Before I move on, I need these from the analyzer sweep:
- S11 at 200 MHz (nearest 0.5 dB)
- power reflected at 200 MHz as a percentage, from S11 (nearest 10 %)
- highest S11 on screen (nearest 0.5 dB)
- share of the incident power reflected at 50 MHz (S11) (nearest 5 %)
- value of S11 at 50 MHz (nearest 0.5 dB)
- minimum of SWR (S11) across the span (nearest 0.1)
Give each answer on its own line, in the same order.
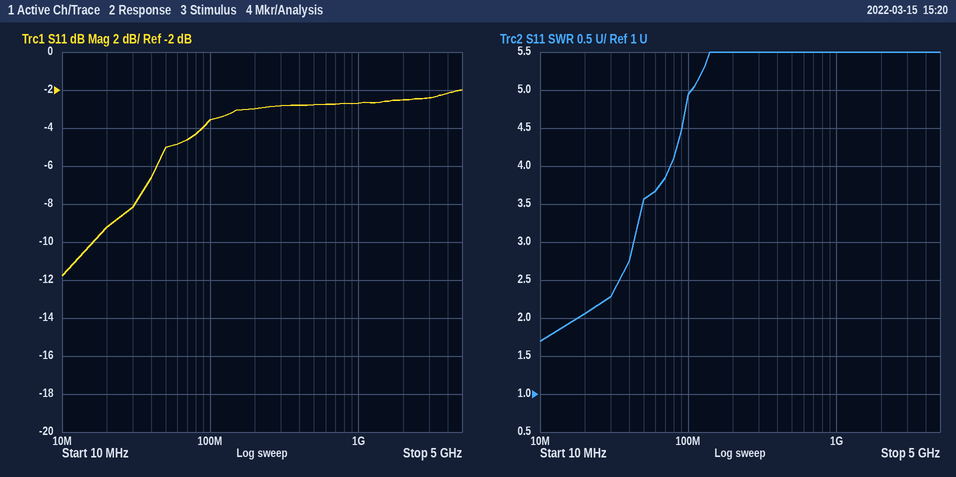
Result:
-3.0 dB
50 %
-2.0 dB
30 %
-5.0 dB
1.7
